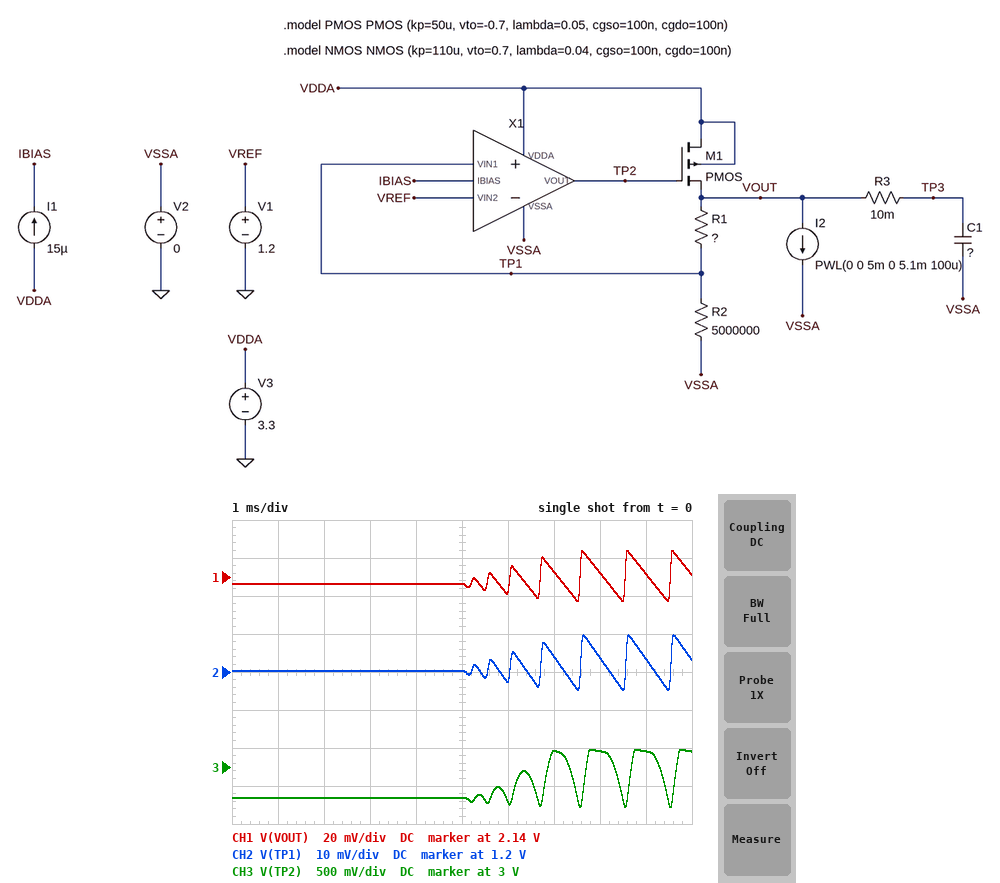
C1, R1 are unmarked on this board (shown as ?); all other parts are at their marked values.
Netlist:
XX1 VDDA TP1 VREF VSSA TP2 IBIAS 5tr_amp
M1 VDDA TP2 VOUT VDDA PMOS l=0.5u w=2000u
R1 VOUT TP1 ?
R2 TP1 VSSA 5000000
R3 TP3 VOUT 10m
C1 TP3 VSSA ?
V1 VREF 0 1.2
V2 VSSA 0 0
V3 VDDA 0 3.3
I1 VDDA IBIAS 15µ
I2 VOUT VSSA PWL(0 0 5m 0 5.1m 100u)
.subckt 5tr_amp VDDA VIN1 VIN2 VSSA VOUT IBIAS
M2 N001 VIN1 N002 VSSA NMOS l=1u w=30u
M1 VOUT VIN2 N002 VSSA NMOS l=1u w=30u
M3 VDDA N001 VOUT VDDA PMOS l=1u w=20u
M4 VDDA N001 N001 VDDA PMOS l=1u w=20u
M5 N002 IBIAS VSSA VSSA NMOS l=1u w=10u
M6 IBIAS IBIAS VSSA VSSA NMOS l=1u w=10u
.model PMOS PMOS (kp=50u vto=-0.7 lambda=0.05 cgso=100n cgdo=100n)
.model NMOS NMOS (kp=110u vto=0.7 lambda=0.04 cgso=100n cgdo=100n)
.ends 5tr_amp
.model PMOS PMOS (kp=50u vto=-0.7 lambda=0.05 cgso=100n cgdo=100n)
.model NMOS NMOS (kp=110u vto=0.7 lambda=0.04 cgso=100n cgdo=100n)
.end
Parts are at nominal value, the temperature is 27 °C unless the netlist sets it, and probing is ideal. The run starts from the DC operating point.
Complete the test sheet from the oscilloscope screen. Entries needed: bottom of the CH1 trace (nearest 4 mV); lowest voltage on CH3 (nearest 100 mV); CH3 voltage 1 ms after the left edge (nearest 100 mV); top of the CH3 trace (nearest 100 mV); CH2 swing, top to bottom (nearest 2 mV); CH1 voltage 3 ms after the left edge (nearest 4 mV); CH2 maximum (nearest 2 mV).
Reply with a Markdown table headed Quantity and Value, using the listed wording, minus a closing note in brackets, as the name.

| Quantity | Value |
|---|---|
| bottom of the CH1 trace | 2.128 V |
| lowest voltage on CH3 | 2.5 V |
| CH3 voltage 1 ms after the left edge | 2.6 V |
| top of the CH3 trace | 3.2 V |
| CH2 swing, top to bottom | 14 mV |
| CH1 voltage 3 ms after the left edge | 2.136 V |
| CH2 maximum | 1.210 V |
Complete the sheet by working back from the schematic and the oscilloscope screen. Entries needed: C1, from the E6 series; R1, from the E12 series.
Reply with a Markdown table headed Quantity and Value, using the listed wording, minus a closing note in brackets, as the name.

| Quantity | Value |
|---|---|
| C1, from the E6 series | 3.3 µF |
| R1, from the E12 series | 3.9 MΩ |
